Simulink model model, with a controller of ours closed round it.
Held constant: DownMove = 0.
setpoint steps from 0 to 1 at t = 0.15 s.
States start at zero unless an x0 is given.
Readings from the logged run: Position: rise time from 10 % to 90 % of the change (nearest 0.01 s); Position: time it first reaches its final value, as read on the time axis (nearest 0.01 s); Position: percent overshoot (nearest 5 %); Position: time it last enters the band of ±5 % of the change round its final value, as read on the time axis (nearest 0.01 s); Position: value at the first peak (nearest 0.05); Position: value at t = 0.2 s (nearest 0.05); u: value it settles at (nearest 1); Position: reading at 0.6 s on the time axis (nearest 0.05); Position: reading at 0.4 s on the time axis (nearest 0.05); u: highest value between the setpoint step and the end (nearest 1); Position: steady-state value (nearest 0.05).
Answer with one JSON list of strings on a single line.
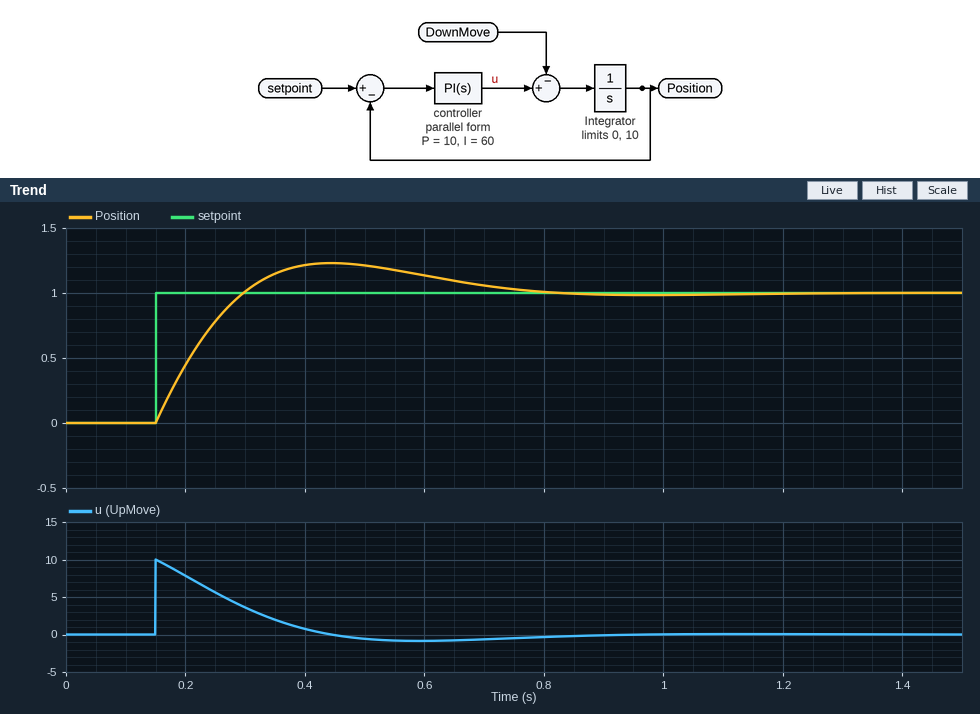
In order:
["0.11 s", "0.30 s", "25 %", "0.71 s", "1.25", "0.45", "0", "1.15", "1.20", "10", "1.00"]
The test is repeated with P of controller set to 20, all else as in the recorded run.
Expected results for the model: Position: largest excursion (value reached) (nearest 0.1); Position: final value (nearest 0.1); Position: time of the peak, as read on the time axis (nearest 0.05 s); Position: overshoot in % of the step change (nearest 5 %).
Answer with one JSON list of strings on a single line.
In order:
["1.1", "1.0", "0.40 s", "10 %"]
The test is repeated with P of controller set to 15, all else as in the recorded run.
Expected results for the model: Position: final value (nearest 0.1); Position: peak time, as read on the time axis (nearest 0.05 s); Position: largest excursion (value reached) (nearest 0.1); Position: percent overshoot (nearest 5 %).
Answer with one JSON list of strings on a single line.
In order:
["1.0", "0.40 s", "1.1", "15 %"]
